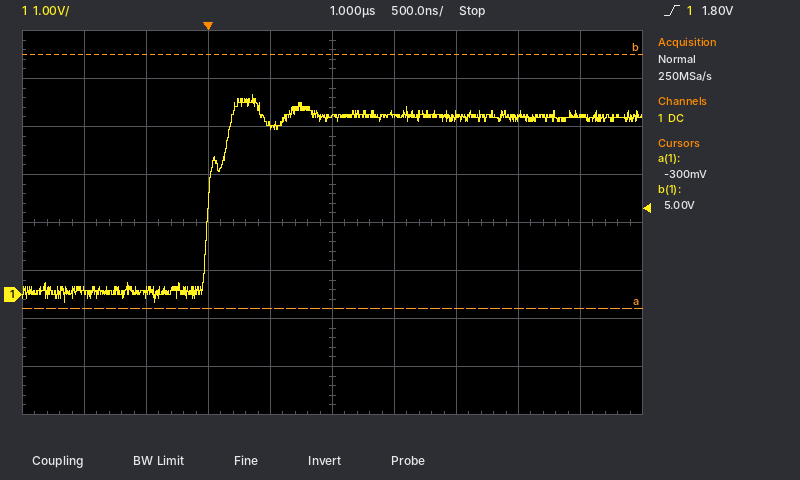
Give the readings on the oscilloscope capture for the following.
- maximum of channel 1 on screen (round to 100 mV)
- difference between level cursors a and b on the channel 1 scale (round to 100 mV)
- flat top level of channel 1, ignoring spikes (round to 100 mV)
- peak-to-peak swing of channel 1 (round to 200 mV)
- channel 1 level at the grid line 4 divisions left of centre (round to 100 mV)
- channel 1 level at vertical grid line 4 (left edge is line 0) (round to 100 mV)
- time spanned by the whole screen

4.2 V
5.3 V
3.7 V
4.4 V
100 mV
3.5 V
5 µs
